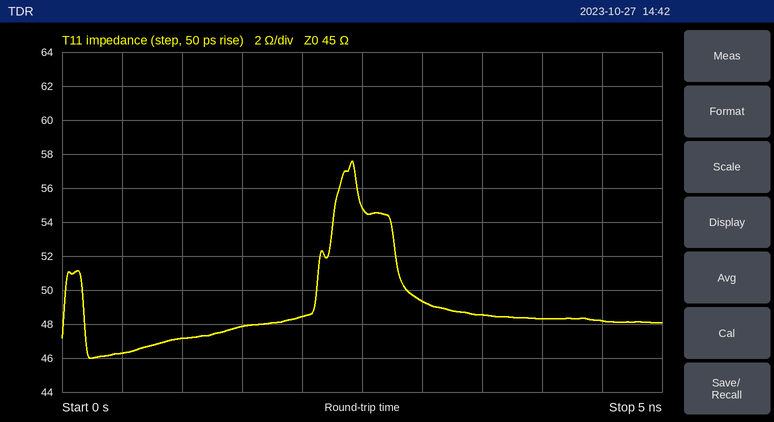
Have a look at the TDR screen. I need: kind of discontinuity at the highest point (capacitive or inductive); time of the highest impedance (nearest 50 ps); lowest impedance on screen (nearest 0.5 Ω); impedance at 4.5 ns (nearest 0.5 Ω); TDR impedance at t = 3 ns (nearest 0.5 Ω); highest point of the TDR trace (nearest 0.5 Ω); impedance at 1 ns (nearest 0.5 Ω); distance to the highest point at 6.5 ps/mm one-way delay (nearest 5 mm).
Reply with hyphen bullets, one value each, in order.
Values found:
- inductive
- 2.40 ns
- 46.0 Ω
- 48.0 Ω
- 49.5 Ω
- 57.5 Ω
- 47.0 Ω
- 185 mm
